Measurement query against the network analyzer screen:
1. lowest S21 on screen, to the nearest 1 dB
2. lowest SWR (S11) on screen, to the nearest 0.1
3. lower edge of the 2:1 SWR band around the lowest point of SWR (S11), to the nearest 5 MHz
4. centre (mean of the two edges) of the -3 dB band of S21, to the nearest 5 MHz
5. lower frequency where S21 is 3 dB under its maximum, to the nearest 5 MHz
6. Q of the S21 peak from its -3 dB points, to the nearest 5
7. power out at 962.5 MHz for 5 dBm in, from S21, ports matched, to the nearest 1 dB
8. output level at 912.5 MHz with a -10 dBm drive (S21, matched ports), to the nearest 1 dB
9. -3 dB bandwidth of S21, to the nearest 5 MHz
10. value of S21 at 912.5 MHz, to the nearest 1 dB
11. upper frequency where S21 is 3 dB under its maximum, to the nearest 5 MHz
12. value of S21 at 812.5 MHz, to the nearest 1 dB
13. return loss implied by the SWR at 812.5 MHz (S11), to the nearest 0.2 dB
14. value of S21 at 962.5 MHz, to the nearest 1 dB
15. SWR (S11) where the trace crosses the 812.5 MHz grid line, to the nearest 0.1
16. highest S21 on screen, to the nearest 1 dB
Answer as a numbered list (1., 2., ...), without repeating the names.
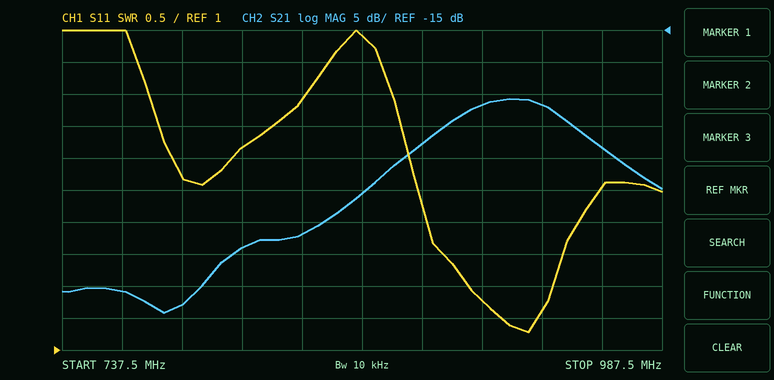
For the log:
1. -59 dB
2. 1.3
3. 905 MHz
4. 925 MHz
5. 900 MHz
6. 20
7. -28 dBm
8. -37 dBm
9. 45 MHz
10. -27 dB
11. 945 MHz
12. -49 dB
13. 4.2 dB
14. -33 dB
15. 4.2
16. -26 dB
